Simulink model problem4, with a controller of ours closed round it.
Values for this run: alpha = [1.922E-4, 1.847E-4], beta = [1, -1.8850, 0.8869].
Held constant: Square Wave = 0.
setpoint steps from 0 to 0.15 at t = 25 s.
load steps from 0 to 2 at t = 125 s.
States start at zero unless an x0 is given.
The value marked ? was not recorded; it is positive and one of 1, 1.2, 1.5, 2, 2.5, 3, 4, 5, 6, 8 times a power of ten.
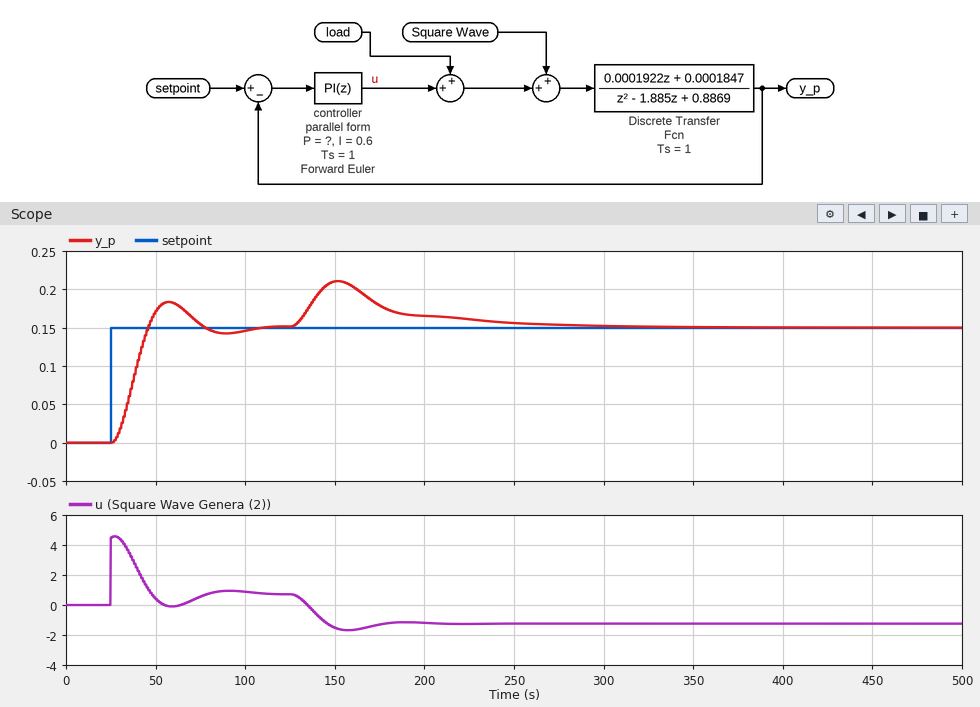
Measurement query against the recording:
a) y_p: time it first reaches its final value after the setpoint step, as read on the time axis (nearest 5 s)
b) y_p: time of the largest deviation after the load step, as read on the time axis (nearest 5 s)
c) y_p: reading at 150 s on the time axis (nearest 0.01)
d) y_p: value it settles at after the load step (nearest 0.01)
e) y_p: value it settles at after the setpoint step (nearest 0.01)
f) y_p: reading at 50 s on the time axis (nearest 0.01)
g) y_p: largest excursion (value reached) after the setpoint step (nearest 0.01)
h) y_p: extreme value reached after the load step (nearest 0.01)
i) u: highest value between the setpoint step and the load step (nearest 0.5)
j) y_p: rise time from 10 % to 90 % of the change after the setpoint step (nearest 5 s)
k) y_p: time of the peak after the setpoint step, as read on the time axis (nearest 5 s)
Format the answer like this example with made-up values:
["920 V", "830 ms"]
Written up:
["45 s", "150 s", "0.21", "0.15", "0.15", "0.17", "0.18", "0.21", "4.5", "15 s", "55 s"]
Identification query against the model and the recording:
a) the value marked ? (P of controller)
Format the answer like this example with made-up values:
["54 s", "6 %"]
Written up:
["30"]
